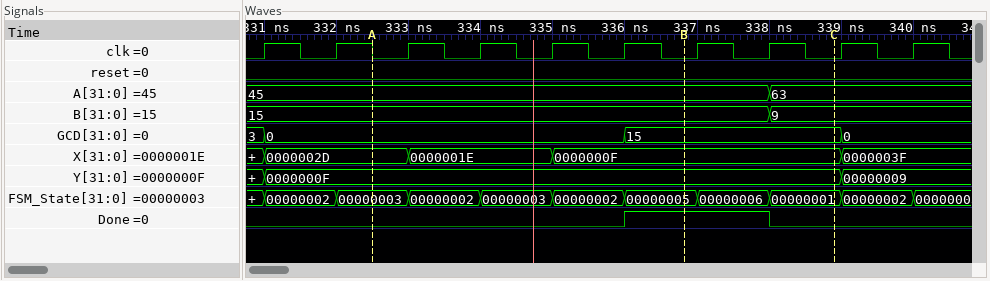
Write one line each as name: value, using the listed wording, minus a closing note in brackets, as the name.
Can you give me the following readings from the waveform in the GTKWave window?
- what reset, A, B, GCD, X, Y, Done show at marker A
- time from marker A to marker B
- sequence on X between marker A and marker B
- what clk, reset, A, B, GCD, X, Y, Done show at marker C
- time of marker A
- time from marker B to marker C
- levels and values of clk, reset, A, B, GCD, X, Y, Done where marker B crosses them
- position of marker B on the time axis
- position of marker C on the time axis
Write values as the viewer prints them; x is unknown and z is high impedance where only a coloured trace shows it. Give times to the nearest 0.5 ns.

what reset, A, B, GCD, X, Y, Done show at marker A: reset=0, A=45, B=15, GCD=0, X=0000002D, Y=0000000F, Done=0
time from marker A to marker B: 4.5 ns
sequence on X between marker A and marker B: 0000002D, 0000001E, 0000000F
what clk, reset, A, B, GCD, X, Y, Done show at marker C: clk=0, reset=0, A=63, B=9, GCD=15, X=0000000F, Y=0000000F, Done=0
time of marker A: 332.5 ns
time from marker B to marker C: 2 ns
levels and values of clk, reset, A, B, GCD, X, Y, Done where marker B crosses them: clk=0, reset=0, A=45, B=15, GCD=15, X=0000000F, Y=0000000F, Done=1
position of marker B on the time axis: 337 ns
position of marker C on the time axis: 339 ns
